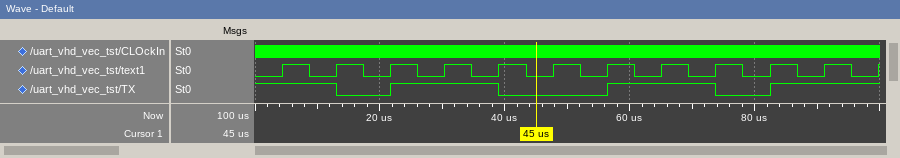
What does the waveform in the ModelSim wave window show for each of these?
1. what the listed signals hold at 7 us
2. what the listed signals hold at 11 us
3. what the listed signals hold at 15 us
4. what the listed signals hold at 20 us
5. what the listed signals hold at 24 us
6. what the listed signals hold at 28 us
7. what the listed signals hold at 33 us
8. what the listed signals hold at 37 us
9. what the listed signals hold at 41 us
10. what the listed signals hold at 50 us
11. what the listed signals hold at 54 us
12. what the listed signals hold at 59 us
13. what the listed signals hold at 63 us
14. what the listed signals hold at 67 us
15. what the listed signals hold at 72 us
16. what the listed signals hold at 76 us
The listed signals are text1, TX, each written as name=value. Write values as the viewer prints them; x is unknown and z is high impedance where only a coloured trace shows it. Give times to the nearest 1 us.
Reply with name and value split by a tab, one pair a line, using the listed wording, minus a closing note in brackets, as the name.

what the listed signals hold at 7 us	text1=1, TX=1
what the listed signals hold at 11 us	text1=0, TX=1
what the listed signals hold at 15 us	text1=1, TX=0
what the listed signals hold at 20 us	text1=0, TX=0
what the listed signals hold at 24 us	text1=1, TX=1
what the listed signals hold at 28 us	text1=0, TX=1
what the listed signals hold at 33 us	text1=1, TX=1
what the listed signals hold at 37 us	text1=0, TX=1
what the listed signals hold at 41 us	text1=1, TX=0
what the listed signals hold at 50 us	text1=1, TX=0
what the listed signals hold at 54 us	text1=0, TX=0
what the listed signals hold at 59 us	text1=1, TX=1
what the listed signals hold at 63 us	text1=0, TX=1
what the listed signals hold at 67 us	text1=1, TX=1
what the listed signals hold at 72 us	text1=0, TX=1
what the listed signals hold at 76 us	text1=1, TX=0
